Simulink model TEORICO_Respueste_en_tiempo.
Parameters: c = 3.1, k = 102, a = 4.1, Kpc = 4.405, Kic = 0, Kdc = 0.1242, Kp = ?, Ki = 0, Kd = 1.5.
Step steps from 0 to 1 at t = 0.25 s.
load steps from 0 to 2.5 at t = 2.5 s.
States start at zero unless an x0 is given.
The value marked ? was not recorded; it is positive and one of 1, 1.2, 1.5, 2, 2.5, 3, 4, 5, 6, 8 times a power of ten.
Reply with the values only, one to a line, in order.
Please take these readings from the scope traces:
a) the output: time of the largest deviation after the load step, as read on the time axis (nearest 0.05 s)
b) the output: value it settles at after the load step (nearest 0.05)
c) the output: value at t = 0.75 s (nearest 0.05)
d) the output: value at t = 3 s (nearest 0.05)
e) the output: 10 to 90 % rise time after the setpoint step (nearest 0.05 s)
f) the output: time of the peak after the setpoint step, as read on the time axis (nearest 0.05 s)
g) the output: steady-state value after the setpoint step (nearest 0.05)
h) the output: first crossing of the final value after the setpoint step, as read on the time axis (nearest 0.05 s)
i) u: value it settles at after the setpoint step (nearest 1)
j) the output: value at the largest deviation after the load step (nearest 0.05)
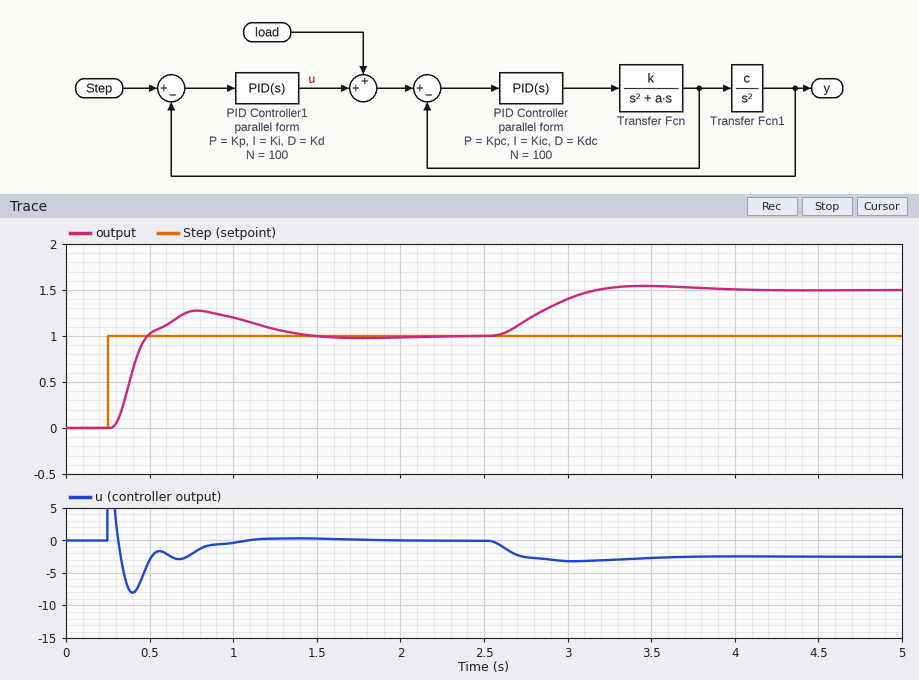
3.45 s
1.50
1.25
1.40
0.15 s
0.80 s
1.00
0.50 s
0
1.55
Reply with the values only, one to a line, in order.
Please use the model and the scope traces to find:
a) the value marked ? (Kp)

5
